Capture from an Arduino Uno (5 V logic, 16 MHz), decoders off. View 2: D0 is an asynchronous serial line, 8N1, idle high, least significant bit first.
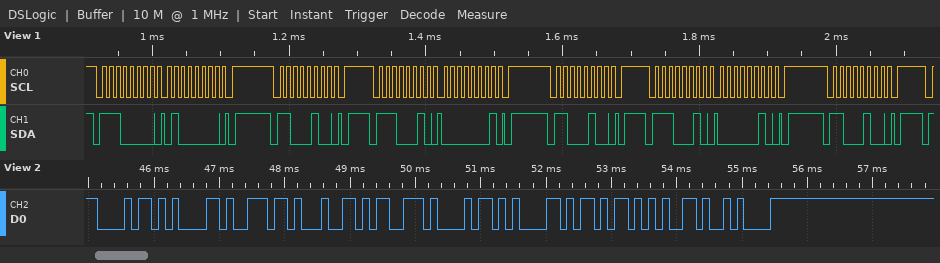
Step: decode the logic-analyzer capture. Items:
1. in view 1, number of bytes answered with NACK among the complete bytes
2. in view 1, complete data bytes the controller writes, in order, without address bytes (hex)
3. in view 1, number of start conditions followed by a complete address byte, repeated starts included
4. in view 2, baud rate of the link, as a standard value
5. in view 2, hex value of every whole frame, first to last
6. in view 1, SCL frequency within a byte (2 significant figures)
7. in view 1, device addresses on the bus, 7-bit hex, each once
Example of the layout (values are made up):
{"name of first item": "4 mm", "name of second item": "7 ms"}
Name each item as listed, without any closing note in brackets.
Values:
{"in view 1, number of bytes answered with NACK among the complete bytes": "0", "in view 1, complete data bytes the controller writes, in order, without address bytes": "40 01 02", "in view 1, number of start conditions followed by a complete address byte, repeated starts included": "6", "in view 2, baud rate of the link, as a standard value": "9600 baud", "in view 2, hex value of every whole frame, first to last": "68 61 6E 64 73 68 61 6B 65 0A", "in view 1, SCL frequency within a byte": "100 kHz", "in view 1, device addresses on the bus, 7-bit hex, each once": "0x70 0x62 0x71"}
